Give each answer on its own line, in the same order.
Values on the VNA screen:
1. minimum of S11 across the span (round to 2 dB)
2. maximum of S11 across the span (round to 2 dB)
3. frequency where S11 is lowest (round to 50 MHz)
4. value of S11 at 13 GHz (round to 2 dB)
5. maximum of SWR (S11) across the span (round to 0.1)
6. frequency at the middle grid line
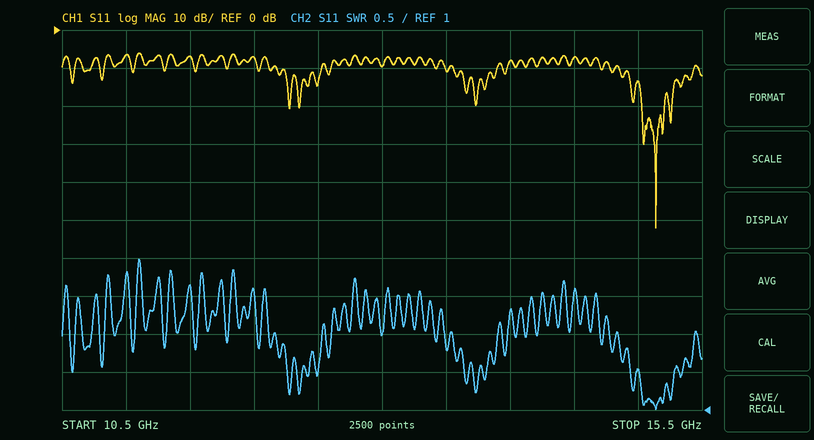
-52 dB
-6 dB
15.15 GHz
-10 dB
3.0
13 GHz
